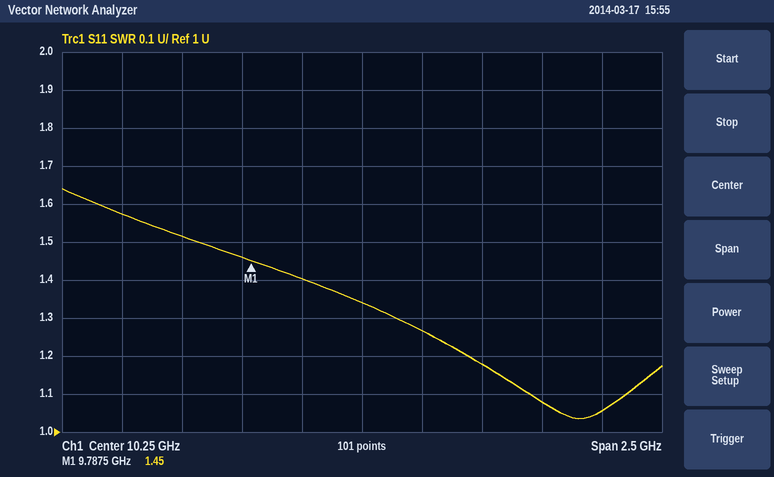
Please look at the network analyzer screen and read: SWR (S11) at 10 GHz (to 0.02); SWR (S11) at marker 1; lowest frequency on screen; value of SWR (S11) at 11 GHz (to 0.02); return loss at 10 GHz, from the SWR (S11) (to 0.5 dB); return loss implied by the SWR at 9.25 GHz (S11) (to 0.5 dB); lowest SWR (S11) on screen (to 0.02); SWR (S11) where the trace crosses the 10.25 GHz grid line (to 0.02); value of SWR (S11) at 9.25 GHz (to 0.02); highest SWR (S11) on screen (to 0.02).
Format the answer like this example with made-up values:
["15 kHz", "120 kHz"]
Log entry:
["1.40", "1.45", "9 GHz", "1.08", "15.5 dB", "13.0 dB", "1.04", "1.34", "1.58", "1.64"]
